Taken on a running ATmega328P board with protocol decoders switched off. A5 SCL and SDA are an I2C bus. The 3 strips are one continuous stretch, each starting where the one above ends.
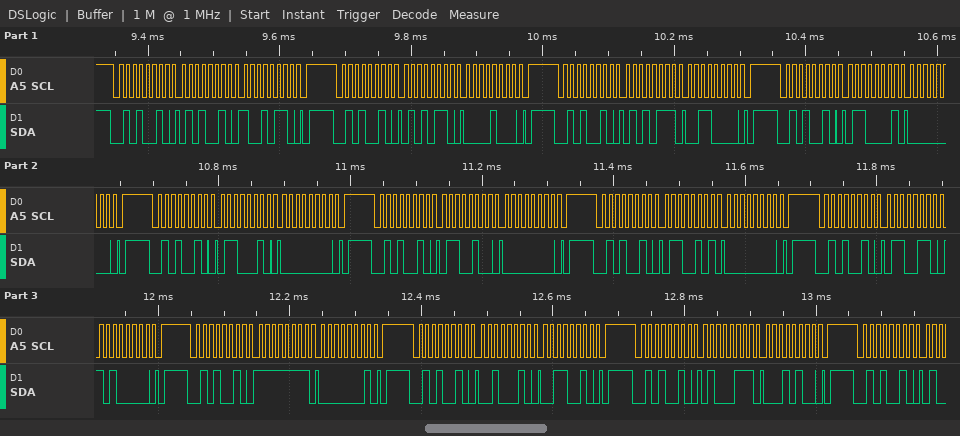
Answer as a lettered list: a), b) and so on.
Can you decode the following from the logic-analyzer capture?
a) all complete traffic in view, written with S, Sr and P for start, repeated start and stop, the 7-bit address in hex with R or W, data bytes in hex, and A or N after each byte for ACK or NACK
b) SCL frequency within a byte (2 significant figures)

a) S 29W A 52 A 96 A P S 29W A 56 A 08 A P S 29W A 57 A 30 A P S 29W A 61 A 00 A P S 29W A 62 A 00 A P S 29W A 64 A 00 A P S 29W A 65 A 00 A P S 29W A 66 A A0 A P S 29W A FF A 01 A P S 29W A 22 A 32 A P S 29W A 47 A 14 A P S 29W A
b) 100 kHz
